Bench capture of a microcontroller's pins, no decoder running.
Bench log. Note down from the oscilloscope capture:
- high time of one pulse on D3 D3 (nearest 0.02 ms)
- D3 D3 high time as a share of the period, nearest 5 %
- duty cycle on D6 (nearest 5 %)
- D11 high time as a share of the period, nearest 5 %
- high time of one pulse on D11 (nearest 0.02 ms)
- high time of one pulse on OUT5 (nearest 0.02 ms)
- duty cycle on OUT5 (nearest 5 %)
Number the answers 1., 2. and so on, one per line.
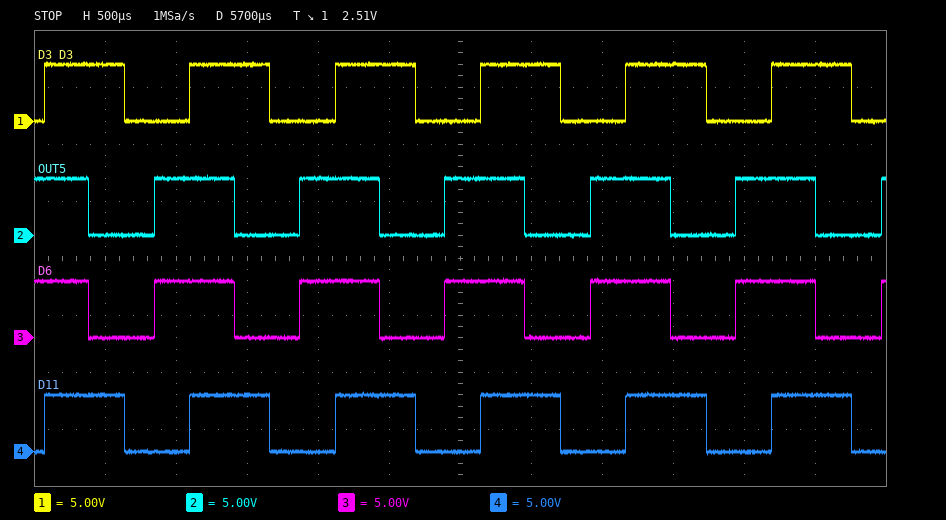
1. 0.56 ms
2. 55 %
3. 55 %
4. 55 %
5. 0.56 ms
6. 0.56 ms
7. 55 %
